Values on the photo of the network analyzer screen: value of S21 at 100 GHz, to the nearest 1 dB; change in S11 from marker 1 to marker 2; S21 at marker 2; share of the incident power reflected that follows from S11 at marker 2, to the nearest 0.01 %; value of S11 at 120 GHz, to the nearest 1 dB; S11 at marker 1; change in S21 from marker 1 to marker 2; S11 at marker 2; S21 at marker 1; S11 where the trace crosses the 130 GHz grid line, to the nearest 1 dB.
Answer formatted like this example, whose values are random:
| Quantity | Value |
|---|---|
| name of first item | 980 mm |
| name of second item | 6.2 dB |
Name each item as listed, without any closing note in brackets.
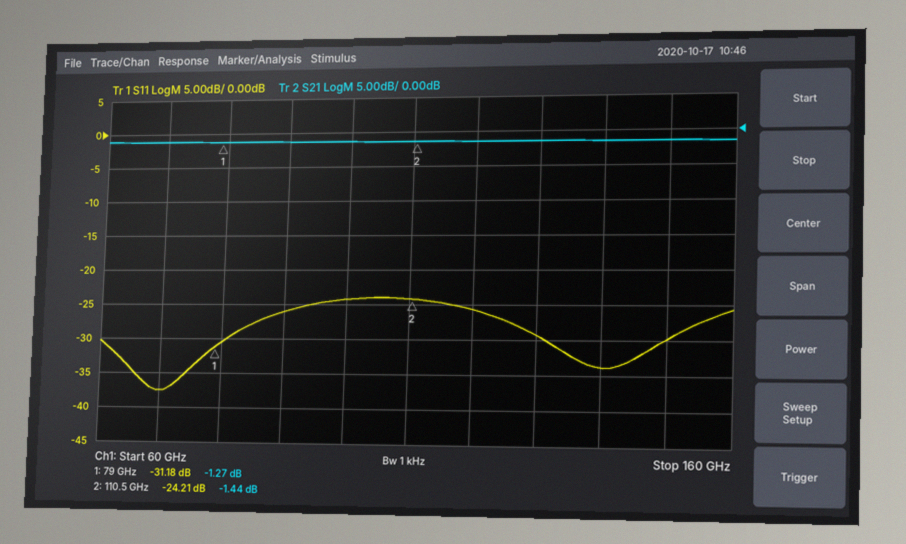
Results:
| Quantity | Value |
|---|---|
| value of S21 at 100 GHz, to the nearest 1 dB | -1 dB |
| change in S11 from marker 1 to marker 2 | 6.97 dB |
| S21 at marker 2 | -1.44 dB |
| share of the incident power reflected that follows from S11 at marker 2, to the nearest 0.01 % | 0.38 % |
| value of S11 at 120 GHz, to the nearest 1 dB | -26 dB |
| S11 at marker 1 | -31.18 dB |
| change in S21 from marker 1 to marker 2 | -0.17 dB |
| S11 at marker 2 | -24.21 dB |
| S21 at marker 1 | -1.27 dB |
| S11 where the trace crosses the 130 GHz grid line, to the nearest 1 dB | -29 dB |
